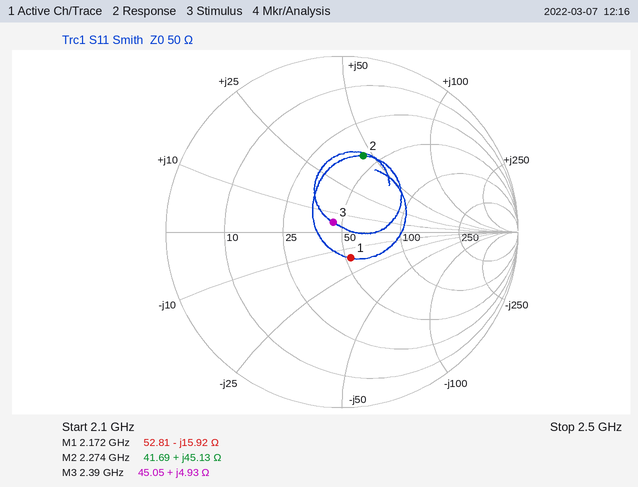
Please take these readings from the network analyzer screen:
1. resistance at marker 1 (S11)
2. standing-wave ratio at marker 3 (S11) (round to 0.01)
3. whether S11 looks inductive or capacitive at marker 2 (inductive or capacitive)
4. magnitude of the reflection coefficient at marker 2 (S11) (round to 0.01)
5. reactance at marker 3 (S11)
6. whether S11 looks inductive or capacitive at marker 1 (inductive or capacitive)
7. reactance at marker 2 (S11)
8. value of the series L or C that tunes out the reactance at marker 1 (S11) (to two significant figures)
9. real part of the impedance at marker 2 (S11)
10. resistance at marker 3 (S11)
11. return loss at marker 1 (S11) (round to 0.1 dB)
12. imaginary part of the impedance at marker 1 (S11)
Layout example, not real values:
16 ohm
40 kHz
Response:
52.81 Ω
1.16
inductive
0.45
+4.93 Ω
capacitive
+45.13 Ω
1.2 nH
41.69 Ω
45.05 Ω
16.2 dB
-15.92 Ω
